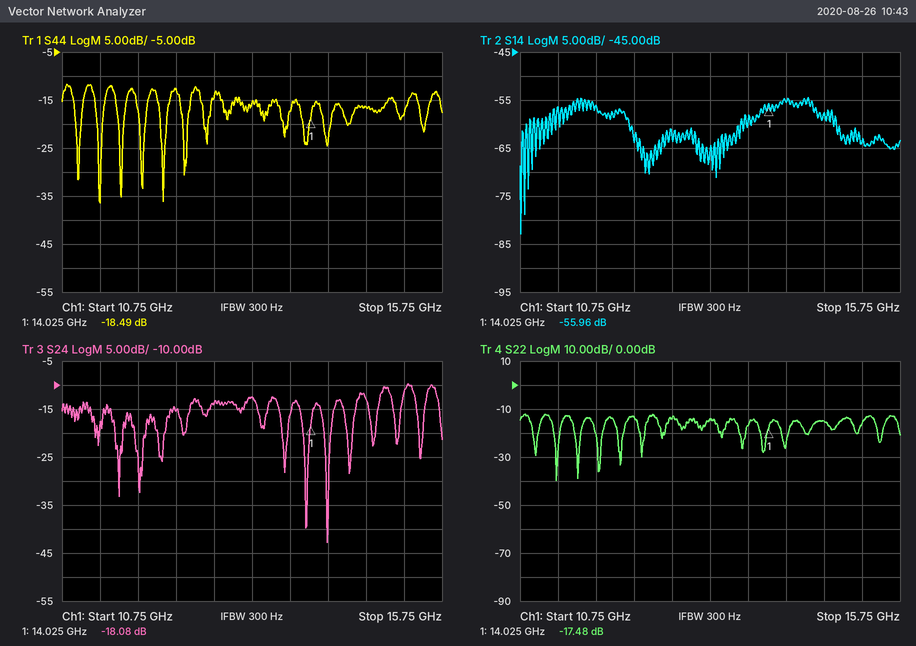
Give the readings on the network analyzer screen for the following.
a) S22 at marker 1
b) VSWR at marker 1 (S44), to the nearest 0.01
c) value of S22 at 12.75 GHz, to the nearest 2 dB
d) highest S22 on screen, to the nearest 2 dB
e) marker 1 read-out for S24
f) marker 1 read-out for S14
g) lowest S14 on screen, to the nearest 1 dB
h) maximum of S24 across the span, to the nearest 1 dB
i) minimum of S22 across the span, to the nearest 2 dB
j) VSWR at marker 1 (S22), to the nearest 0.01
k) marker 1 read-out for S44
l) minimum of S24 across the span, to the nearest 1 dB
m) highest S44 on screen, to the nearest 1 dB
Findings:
-17.48 dB
1.27
-14 dB
-12 dB
-18.08 dB
-55.96 dB
-83 dB
-10 dB
-40 dB
1.31
-18.49 dB
-43 dB
-12 dB
